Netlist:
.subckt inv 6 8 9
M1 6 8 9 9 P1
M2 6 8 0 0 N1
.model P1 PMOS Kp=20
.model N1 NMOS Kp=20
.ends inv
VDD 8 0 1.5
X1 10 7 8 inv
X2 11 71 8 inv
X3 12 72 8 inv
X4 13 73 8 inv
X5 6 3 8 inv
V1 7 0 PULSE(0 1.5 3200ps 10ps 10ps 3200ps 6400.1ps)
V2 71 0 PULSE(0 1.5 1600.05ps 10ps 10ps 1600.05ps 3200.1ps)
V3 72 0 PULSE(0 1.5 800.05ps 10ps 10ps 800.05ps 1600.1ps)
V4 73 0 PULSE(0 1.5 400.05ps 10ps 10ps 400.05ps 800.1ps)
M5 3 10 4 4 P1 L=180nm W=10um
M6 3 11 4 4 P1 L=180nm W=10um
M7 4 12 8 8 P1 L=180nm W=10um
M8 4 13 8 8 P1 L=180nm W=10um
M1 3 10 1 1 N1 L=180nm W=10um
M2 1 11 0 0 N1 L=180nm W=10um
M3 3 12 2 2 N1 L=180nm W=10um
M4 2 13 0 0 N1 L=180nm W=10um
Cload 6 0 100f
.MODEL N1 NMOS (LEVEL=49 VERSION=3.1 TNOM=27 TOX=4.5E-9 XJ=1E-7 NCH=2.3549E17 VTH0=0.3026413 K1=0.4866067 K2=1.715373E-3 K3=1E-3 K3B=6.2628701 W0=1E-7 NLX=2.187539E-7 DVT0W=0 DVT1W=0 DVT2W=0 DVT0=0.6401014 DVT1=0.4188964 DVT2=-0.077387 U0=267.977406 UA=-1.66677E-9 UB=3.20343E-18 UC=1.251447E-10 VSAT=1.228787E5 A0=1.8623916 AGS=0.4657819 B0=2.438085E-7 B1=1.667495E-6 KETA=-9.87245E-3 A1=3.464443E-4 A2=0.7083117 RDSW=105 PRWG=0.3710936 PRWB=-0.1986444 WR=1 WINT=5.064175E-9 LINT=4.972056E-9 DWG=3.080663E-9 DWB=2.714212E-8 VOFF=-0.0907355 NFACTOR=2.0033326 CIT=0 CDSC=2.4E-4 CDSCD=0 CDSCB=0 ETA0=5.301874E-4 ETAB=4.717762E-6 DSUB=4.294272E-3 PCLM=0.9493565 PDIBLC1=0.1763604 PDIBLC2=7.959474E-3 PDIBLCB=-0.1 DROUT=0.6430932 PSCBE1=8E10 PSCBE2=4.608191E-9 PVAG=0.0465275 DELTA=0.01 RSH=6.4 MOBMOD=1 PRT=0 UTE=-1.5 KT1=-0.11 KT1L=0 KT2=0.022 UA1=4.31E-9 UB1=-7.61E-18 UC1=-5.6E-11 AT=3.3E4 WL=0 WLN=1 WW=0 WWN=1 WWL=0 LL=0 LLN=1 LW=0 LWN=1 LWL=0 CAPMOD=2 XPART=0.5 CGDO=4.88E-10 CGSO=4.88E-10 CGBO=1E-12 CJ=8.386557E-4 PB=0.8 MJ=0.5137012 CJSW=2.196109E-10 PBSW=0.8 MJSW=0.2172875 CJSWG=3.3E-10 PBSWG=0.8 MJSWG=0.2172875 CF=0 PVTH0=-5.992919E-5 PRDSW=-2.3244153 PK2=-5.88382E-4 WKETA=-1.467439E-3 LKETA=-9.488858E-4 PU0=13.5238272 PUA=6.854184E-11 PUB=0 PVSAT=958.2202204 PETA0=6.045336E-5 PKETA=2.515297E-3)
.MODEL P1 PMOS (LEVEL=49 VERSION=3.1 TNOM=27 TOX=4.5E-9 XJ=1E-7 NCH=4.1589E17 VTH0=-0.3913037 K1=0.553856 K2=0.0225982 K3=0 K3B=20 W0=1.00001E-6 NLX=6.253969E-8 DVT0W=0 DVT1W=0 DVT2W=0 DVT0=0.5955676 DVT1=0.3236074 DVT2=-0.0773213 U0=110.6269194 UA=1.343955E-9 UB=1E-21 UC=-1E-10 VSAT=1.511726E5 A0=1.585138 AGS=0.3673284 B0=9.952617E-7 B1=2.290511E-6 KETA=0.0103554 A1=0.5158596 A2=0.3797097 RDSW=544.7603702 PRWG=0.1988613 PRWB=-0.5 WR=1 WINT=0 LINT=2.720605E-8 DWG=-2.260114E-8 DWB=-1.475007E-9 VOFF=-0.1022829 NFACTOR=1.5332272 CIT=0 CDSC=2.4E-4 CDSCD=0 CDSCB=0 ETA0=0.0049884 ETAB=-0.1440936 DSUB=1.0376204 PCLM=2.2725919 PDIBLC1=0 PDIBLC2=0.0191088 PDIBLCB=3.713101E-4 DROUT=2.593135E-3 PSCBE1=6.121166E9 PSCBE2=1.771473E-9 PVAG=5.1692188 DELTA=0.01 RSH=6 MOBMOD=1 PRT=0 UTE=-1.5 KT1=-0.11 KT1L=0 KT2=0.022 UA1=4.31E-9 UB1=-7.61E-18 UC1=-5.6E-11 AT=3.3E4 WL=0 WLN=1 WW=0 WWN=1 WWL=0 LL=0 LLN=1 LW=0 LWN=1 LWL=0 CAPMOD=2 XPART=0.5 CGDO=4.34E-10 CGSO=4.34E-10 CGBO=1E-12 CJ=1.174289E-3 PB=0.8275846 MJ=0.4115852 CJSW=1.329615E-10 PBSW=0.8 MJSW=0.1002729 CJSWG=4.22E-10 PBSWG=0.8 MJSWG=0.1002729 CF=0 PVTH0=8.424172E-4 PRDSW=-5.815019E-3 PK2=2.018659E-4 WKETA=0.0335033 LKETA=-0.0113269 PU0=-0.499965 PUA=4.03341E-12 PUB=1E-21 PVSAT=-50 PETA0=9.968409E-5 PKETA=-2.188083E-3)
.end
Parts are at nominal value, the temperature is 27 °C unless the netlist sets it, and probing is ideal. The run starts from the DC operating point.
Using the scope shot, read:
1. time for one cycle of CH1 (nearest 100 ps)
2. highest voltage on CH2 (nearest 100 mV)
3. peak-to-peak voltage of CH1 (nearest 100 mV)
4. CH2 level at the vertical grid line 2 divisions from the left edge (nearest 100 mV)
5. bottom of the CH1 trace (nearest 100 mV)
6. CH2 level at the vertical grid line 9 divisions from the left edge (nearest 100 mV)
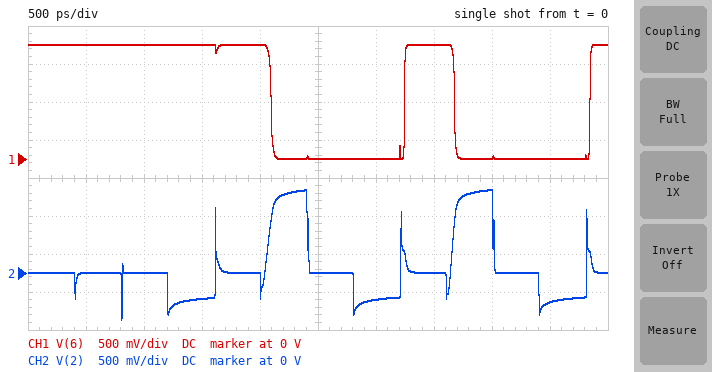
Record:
1.6 ns
1.1 V
1.5 V
0 V
0 V
-400 mV
